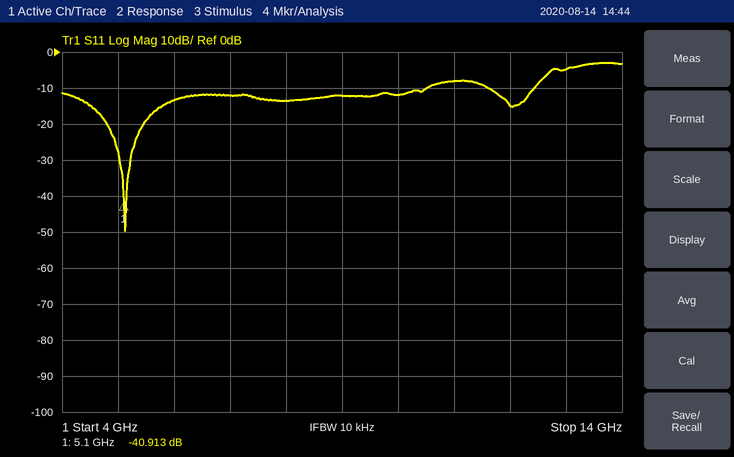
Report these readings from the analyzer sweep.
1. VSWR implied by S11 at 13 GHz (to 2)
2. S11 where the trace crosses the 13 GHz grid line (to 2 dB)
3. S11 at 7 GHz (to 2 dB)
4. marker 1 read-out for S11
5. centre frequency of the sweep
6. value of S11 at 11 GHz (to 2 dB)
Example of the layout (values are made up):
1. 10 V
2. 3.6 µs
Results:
1. 4
2. -4 dB
3. -12 dB
4. -40.913 dB
5. 9 GHz
6. -8 dB
